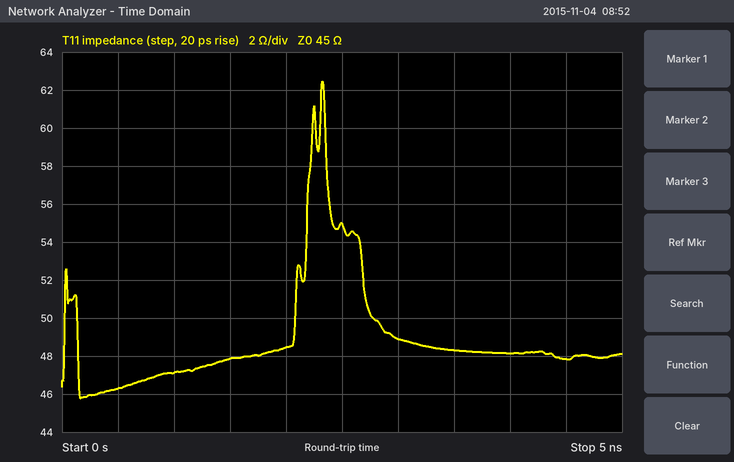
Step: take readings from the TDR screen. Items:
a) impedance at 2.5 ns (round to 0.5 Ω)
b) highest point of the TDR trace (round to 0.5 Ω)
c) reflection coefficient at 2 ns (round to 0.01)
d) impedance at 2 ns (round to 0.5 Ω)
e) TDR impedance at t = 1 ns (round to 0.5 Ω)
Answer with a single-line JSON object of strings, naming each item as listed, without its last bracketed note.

{"impedance at 2.5 ns": "55.0 Ω", "highest point of the TDR trace": "62.5 Ω", "reflection coefficient at 2 ns": "+0.04", "impedance at 2 ns": "48.5 Ω", "TDR impedance at t = 1 ns": "47.0 Ω"}
